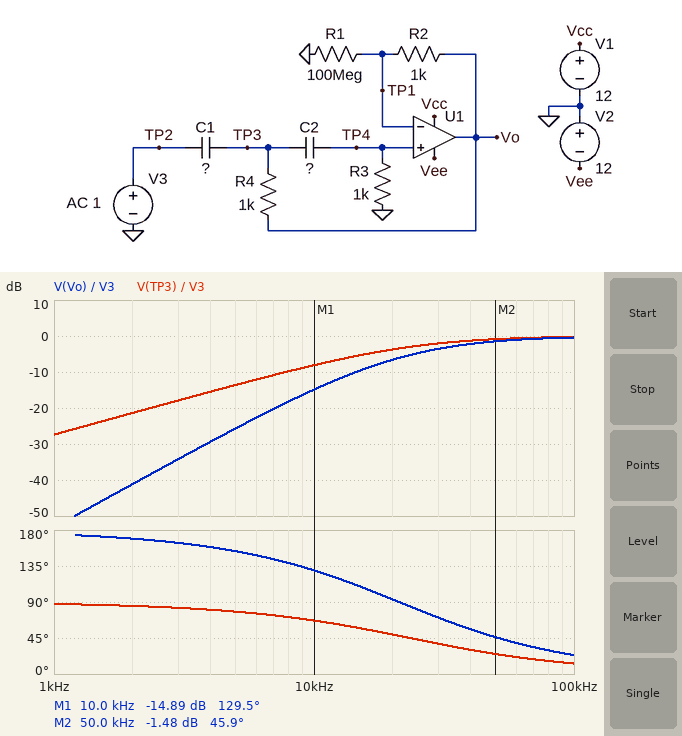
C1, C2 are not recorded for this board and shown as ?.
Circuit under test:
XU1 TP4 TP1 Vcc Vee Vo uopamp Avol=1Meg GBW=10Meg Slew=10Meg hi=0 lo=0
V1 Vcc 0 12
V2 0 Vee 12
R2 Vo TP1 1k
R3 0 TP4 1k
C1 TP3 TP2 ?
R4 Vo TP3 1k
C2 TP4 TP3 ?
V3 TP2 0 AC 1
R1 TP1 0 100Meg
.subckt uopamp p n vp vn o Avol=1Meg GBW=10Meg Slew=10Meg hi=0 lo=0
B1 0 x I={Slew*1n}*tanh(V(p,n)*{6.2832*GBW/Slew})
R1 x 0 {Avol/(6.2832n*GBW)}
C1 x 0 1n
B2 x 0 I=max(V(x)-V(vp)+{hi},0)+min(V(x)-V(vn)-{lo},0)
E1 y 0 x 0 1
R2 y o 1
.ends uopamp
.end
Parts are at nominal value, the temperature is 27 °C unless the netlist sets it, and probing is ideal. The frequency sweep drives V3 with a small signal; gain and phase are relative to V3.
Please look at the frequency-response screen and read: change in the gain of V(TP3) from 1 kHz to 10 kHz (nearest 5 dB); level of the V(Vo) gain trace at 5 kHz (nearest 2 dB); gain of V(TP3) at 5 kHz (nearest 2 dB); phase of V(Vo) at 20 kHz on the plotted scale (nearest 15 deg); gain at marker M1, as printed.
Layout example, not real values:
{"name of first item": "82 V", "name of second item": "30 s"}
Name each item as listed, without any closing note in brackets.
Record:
{"change in the gain of V(TP3) from 1 kHz to 10 kHz": "20 dB", "level of the V(Vo) gain trace at 5 kHz": "-26 dB", "gain of V(TP3) at 5 kHz": "-14 dB", "phase of V(Vo) at 20 kHz on the plotted scale": "90 deg", "gain at marker M1, as printed": "-14.89 dB"}
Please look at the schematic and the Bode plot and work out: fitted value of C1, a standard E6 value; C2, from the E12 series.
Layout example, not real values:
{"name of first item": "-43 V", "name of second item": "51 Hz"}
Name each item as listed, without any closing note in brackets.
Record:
{"fitted value of C1, a standard E6 value": "6.8 nF", "C2, from the E12 series": "8.2 nF"}
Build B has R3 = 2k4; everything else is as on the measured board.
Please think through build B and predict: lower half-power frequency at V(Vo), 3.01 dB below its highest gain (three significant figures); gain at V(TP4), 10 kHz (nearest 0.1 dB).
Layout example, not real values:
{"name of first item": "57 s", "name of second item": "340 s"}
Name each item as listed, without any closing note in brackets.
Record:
{"lower half-power frequency at V(Vo), 3.01 dB below its highest gain": "12.8 kHz", "gain at V(TP4), 10 kHz": "-6.0 dB"}
